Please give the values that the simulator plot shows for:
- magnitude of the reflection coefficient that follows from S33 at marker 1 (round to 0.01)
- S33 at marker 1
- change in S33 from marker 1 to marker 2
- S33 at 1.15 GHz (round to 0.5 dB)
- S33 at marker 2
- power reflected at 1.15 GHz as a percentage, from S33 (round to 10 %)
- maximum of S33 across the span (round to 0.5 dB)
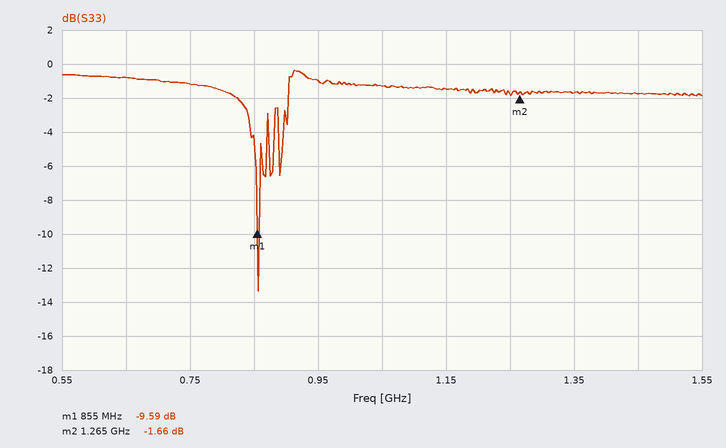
0.33
-9.59 dB
7.93 dB
-1.5 dB
-1.66 dB
70 %
-0.5 dB
